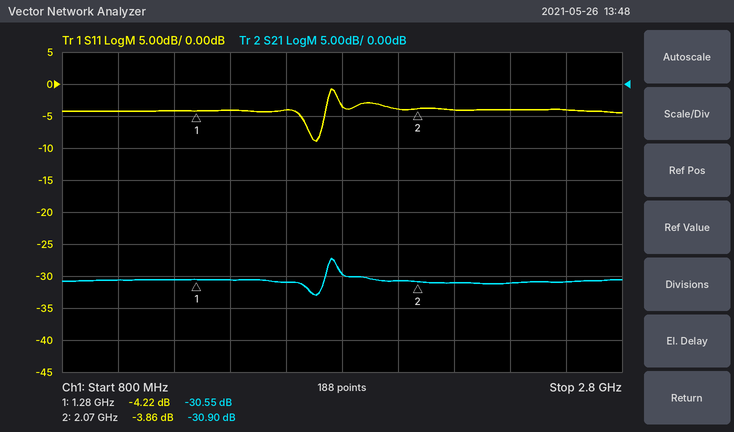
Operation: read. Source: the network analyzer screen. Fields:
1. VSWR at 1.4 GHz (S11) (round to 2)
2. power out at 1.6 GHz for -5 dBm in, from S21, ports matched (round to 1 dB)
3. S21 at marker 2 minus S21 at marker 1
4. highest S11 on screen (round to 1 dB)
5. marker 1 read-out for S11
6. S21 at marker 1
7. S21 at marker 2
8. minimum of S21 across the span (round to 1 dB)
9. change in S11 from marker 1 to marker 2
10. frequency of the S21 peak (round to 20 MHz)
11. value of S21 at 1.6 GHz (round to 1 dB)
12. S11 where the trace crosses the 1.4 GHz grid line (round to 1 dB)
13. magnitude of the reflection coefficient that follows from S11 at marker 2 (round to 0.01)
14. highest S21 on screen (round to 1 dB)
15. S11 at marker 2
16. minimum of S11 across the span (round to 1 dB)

4
-36 dBm
-0.35 dB
-1 dB
-4.22 dB
-30.55 dB
-30.90 dB
-33 dB
0.36 dB
1.76 GHz
-31 dB
-4 dB
0.64
-27 dB
-3.86 dB
-9 dB
